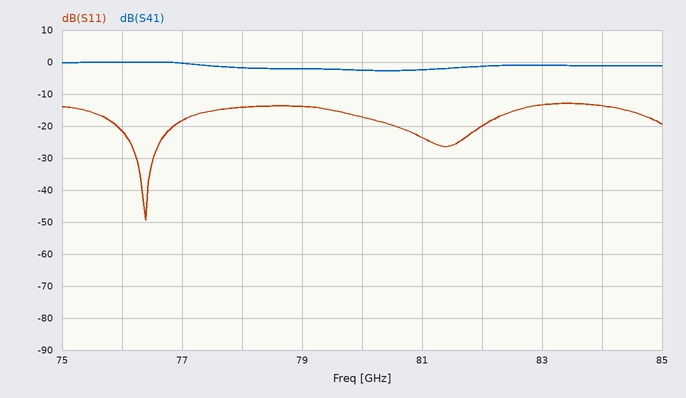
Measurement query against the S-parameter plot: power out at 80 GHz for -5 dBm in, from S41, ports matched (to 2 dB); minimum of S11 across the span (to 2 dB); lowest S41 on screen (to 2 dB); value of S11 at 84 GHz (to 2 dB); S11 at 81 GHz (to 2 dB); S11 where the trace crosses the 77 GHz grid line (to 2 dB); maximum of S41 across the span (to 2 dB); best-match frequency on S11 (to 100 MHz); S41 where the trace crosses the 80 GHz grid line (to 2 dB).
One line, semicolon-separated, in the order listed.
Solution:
-8 dBm; -50 dB; -2 dB; -14 dB; -24 dB; -18 dB; 0 dB; 76.4 GHz; -2 dB
